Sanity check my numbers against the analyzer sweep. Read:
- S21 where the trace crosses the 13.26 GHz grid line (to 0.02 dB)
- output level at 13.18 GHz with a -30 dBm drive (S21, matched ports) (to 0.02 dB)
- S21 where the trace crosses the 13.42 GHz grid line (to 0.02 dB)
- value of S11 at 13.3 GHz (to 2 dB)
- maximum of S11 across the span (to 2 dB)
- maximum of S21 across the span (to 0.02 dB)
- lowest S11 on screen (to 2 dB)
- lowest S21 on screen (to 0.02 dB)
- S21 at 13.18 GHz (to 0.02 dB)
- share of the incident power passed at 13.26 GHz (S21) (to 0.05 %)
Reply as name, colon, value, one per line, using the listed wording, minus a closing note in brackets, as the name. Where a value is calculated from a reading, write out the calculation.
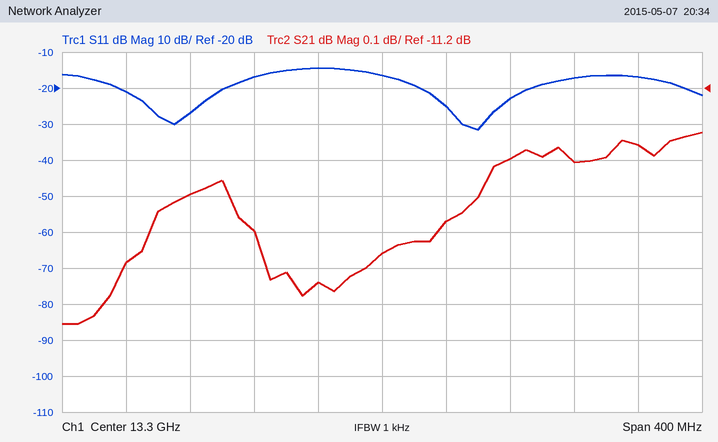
S21 where the trace crosses the 13.26 GHz grid line: -11.74 dB
output level at 13.18 GHz with a -30 dBm drive (S21, matched ports): -30 dBm + (-11.50 dB) = -41.50 dBm
S21 where the trace crosses the 13.42 GHz grid line: -11.40 dB
value of S11 at 13.3 GHz: -16 dB
maximum of S11 across the span: -14 dB
maximum of S21 across the span: -11.32 dB
lowest S11 on screen: -32 dB
lowest S21 on screen: -11.86 dB
S21 at 13.18 GHz: -11.50 dB
share of the incident power passed at 13.26 GHz (S21): 10^(-11.74/10) ≈ 6.70 %
